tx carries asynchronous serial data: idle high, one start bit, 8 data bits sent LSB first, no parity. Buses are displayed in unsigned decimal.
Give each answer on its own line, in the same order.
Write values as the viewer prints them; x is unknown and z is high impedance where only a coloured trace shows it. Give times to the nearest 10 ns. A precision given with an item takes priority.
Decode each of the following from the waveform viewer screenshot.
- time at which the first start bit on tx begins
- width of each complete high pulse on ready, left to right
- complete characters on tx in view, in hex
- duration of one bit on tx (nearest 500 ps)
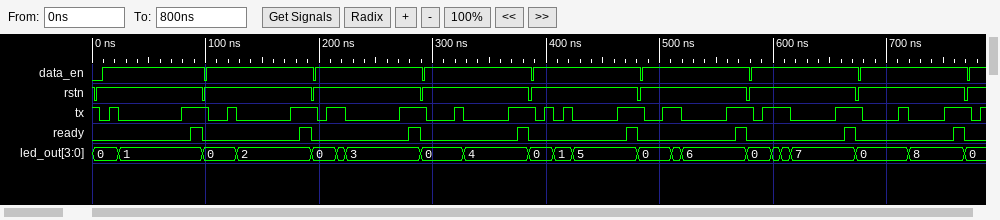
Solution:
10 ns
10 ns, 10 ns, 10 ns, 10 ns, 10 ns, 10 ns, 10 ns, 10 ns
01, 02, 03, 04, 05, 06, 07, 08
8000 ps
